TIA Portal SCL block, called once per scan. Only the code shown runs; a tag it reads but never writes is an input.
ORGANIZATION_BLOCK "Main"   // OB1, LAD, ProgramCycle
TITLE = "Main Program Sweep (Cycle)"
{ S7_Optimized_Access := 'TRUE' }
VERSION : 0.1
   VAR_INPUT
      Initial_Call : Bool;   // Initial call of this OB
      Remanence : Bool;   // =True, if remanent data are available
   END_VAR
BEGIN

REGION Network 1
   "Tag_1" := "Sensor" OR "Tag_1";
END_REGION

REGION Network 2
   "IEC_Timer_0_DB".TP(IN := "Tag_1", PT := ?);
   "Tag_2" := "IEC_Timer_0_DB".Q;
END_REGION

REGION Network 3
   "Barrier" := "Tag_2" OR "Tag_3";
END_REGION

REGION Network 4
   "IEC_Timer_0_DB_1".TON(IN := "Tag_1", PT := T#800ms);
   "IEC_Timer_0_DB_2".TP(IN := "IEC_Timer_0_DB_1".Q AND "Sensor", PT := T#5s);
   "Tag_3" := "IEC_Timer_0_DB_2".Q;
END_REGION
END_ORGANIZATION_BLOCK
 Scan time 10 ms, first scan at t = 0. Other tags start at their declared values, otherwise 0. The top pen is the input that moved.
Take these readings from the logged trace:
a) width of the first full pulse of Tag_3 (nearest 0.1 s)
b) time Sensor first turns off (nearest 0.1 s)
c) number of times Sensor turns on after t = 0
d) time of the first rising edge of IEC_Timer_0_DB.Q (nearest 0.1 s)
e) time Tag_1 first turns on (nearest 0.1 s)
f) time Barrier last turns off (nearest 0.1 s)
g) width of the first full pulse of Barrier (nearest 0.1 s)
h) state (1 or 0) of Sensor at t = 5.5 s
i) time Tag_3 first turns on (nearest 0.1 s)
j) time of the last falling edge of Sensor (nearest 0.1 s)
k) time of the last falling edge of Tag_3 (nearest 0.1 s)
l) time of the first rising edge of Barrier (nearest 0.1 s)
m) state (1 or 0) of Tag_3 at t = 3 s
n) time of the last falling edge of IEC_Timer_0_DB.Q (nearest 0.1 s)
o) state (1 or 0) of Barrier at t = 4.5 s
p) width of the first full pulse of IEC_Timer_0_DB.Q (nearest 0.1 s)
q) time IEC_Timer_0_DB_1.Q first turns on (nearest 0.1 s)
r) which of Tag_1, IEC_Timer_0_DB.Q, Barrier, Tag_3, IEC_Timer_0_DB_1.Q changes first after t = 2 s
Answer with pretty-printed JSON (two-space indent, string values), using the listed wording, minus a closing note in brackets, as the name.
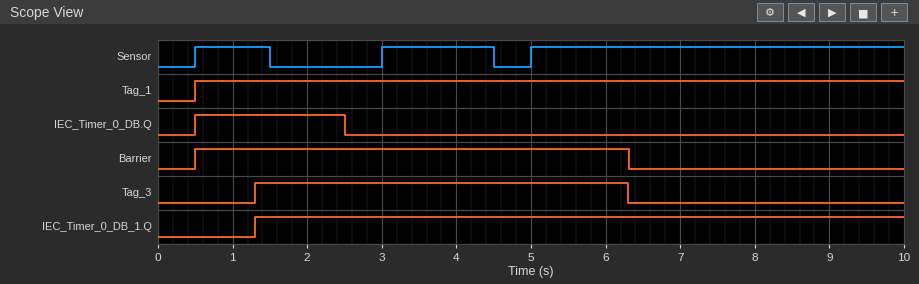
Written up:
{
  "width of the first full pulse of Tag_3": "5.0 s",
  "time Sensor first turns off": "1.5 s",
  "number of times Sensor turns on after t = 0": "3",
  "time of the first rising edge of IEC_Timer_0_DB.Q": "0.5 s",
  "time Tag_1 first turns on": "0.5 s",
  "time Barrier last turns off": "6.3 s",
  "width of the first full pulse of Barrier": "5.8 s",
  "state (1 or 0) of Sensor at t = 5.5 s": "1",
  "time Tag_3 first turns on": "1.3 s",
  "time of the last falling edge of Sensor": "4.5 s",
  "time of the last falling edge of Tag_3": "6.3 s",
  "time of the first rising edge of Barrier": "0.5 s",
  "state (1 or 0) of Tag_3 at t = 3 s": "1",
  "time of the last falling edge of IEC_Timer_0_DB.Q": "2.5 s",
  "state (1 or 0) of Barrier at t = 4.5 s": "1",
  "width of the first full pulse of IEC_Timer_0_DB.Q": "2.0 s",
  "time IEC_Timer_0_DB_1.Q first turns on": "1.3 s",
  "which of Tag_1, IEC_Timer_0_DB.Q, Barrier, Tag_3, IEC_Timer_0_DB_1.Q changes first after t = 2 s": "IEC_Timer_0_DB.Q"
}
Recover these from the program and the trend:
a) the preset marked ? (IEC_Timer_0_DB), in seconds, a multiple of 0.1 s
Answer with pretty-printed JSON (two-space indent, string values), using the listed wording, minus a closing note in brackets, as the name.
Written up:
{
  "the preset marked ? (IEC_Timer_0_DB), in seconds, a multiple of 0.1 s": "2.0 s"
}
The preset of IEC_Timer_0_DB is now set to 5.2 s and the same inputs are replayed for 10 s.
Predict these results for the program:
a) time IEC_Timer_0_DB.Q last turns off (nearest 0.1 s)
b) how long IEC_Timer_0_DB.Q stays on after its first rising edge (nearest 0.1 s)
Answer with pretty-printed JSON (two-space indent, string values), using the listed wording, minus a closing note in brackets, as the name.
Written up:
{
  "time IEC_Timer_0_DB.Q last turns off": "5.7 s",
  "how long IEC_Timer_0_DB.Q stays on after its first rising edge": "5.2 s"
}
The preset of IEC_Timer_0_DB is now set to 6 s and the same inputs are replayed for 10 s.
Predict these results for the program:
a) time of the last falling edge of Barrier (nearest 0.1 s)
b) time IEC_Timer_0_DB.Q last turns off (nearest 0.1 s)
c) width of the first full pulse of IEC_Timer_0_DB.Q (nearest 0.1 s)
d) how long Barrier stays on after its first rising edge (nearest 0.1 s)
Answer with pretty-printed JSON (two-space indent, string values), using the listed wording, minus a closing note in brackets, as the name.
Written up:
{
  "time of the last falling edge of Barrier": "6.5 s",
  "time IEC_Timer_0_DB.Q last turns off": "6.5 s",
  "width of the first full pulse of IEC_Timer_0_DB.Q": "6.0 s",
  "how long Barrier stays on after its first rising edge": "6.0 s"
}
